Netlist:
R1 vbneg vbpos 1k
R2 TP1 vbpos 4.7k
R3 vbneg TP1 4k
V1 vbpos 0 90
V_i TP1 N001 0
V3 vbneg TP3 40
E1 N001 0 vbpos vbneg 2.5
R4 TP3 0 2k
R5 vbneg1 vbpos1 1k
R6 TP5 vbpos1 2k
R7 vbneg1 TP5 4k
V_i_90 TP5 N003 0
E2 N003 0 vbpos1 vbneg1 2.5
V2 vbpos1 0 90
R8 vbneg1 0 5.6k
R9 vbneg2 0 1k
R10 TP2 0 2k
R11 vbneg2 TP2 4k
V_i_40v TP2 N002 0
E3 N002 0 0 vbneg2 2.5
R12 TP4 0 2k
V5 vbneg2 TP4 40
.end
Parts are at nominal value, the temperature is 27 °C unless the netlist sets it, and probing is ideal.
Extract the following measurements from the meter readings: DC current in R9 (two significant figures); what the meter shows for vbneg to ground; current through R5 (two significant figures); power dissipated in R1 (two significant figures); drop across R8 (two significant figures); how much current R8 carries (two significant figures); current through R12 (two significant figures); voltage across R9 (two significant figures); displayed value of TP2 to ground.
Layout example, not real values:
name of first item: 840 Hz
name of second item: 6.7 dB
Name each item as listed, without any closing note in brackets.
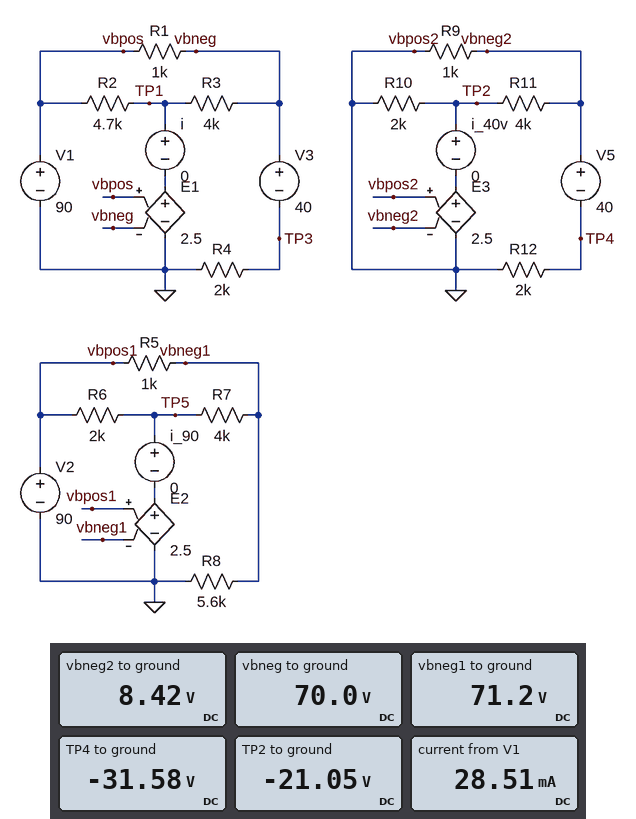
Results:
DC current in R9: 8.4 mA
what the meter shows for vbneg to ground: 70.0 V
current through R5: 19 mA
power dissipated in R1: 400 mW
drop across R8: 71 V
how much current R8 carries: 13 mA
current through R12: 16 mA
voltage across R9: 8.4 V
displayed value of TP2 to ground: -21.05 V
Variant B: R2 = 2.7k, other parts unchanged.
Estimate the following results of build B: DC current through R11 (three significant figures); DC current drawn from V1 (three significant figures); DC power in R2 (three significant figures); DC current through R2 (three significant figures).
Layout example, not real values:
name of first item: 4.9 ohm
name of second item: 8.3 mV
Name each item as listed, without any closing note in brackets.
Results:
DC current through R11: 7.37 mA
DC current drawn from V1: 34.8 mA
DC power in R2: 593 mW
DC current through R2: 14.8 mA
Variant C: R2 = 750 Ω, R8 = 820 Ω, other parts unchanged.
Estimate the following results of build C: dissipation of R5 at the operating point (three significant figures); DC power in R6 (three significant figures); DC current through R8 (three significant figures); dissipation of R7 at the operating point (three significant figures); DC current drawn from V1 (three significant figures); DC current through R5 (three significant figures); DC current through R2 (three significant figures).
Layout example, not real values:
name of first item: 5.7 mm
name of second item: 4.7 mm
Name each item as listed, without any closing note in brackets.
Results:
dissipation of R5 at the operating point: 1.83 W
DC power in R6: 142 mW
DC current through R8: 57.6 mA
dissipation of R7 at the operating point: 888 mW
DC current drawn from V1: 73.3 mA
DC current through R5: 42.7 mA
DC current through R2: 53.3 mA
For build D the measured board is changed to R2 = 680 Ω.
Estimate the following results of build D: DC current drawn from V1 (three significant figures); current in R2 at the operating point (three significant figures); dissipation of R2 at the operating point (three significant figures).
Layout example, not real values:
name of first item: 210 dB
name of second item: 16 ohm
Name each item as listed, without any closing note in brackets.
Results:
DC current drawn from V1: 78.8 mA
current in R2 at the operating point: 58.8 mA
dissipation of R2 at the operating point: 2.35 W
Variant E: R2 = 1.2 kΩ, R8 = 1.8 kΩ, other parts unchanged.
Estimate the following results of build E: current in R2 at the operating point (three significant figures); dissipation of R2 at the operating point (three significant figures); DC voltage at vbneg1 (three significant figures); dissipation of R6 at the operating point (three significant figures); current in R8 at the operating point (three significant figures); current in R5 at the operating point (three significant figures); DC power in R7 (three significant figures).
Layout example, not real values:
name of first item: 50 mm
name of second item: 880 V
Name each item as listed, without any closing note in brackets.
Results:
current in R2 at the operating point: 33.3 mA
dissipation of R2 at the operating point: 1.33 W
DC voltage at vbneg1: 60.2 V
dissipation of R6 at the operating point: 119 mW
current in R8 at the operating point: 33.4 mA
current in R5 at the operating point: 29.8 mA
DC power in R7: 51.8 mW
